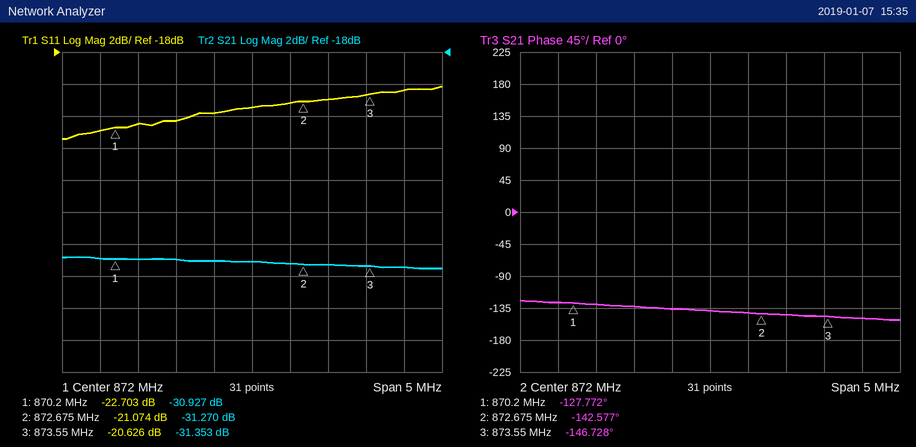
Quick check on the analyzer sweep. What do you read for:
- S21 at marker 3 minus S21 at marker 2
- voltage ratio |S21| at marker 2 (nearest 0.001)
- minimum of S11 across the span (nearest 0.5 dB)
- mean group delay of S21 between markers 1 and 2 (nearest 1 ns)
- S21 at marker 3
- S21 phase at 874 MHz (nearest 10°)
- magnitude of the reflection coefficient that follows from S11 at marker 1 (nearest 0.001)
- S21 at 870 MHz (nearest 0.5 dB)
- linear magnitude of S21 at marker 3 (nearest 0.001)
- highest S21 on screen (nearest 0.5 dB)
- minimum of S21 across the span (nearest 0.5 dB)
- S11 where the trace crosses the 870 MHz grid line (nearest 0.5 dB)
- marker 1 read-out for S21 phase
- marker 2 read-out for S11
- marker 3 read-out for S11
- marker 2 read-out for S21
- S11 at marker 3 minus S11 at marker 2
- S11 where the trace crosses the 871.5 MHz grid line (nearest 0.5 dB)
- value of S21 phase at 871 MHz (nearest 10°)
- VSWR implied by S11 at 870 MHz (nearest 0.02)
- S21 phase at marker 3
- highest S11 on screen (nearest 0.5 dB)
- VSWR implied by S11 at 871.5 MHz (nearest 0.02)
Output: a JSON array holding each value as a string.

["-0.083 dB", "0.027", "-23.5 dB", "17 ns", "-31.353 dB", "-150°", "0.073", "-31.0 dB", "0.027", "-31.0 dB", "-31.5 dB", "-23.0 dB", "-127.772°", "-21.074 dB", "-20.626 dB", "-31.270 dB", "0.448 dB", "-22.0 dB", "-130°", "1.16", "-146.728°", "-20.0 dB", "1.18"]
